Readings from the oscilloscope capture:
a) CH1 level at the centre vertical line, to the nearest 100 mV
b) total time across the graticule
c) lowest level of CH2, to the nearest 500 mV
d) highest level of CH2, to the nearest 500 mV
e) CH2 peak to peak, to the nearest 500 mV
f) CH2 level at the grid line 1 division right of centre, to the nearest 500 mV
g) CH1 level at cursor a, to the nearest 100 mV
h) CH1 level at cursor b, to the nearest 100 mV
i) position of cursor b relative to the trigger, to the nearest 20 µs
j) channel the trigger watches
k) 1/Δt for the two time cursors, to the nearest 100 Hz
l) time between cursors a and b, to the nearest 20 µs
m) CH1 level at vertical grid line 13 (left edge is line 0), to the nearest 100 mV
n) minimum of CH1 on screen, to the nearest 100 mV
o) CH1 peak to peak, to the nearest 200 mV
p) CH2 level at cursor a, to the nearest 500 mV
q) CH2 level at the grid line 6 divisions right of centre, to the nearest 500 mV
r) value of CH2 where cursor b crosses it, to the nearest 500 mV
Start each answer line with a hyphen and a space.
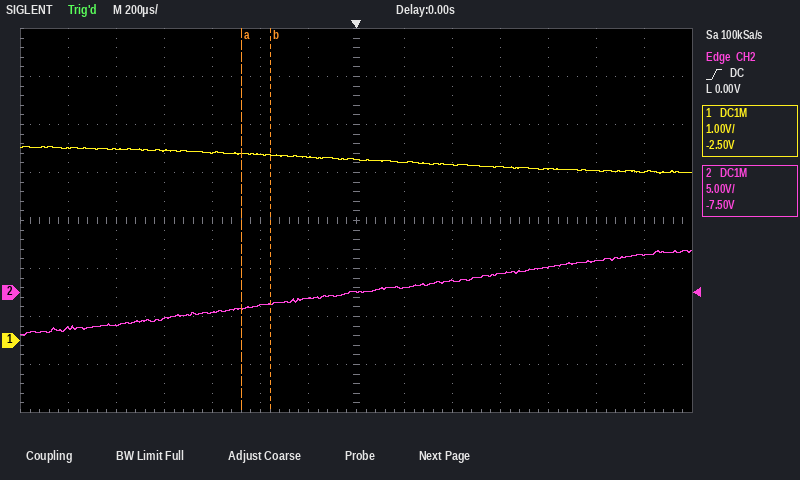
- 3.8 V
- 2.8 ms
- -4.5 V
- 4.5 V
- 9.0 V
- 500 mV
- 3.9 V
- 3.9 V
- -360 µs
- CH2
- 8.3 kHz
- 120 µs
- 3.5 V
- 3.5 V
- 600 mV
- -1.5 V
- 4.0 V
- -1.0 V
